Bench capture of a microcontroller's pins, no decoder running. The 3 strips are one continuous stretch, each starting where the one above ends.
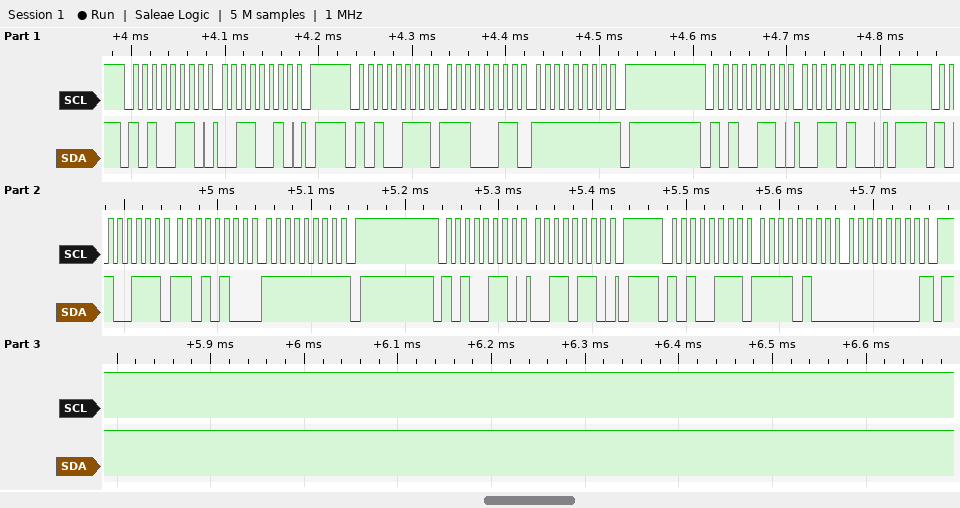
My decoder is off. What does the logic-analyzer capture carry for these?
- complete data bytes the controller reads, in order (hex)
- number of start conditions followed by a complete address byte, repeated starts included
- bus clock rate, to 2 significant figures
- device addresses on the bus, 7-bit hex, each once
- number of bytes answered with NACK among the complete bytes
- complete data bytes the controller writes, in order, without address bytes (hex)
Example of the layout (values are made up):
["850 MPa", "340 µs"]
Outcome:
["E3 FF D4 FF F4 00", "6", "100 kHz", "0x53", "3", "32 34 36"]
